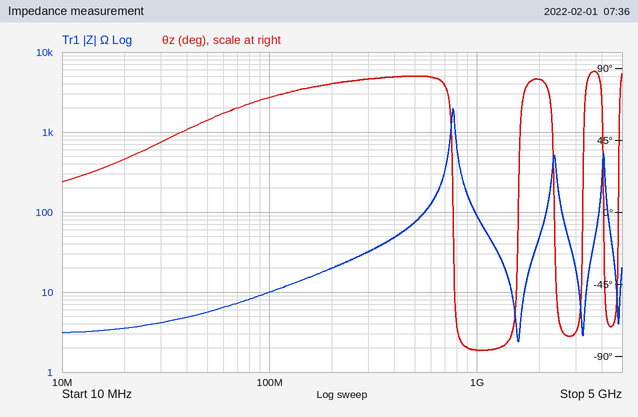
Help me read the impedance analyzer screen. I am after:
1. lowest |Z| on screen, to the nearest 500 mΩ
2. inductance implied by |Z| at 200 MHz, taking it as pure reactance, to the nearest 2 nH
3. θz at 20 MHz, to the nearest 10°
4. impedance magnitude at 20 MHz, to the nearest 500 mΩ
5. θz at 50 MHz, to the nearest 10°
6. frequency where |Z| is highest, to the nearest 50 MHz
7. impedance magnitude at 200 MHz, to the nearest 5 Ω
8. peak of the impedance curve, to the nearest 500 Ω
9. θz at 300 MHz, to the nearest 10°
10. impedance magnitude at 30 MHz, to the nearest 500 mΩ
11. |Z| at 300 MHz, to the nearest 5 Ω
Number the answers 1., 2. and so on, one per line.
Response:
1. 2.5 Ω
2. 16 nH
3. 30°
4. 3.5 Ω
5. 60°
6. 750 MHz
7. 20 Ω
8. 2.0 kΩ
9. 80°
10. 4.0 Ω
11. 30 Ω
